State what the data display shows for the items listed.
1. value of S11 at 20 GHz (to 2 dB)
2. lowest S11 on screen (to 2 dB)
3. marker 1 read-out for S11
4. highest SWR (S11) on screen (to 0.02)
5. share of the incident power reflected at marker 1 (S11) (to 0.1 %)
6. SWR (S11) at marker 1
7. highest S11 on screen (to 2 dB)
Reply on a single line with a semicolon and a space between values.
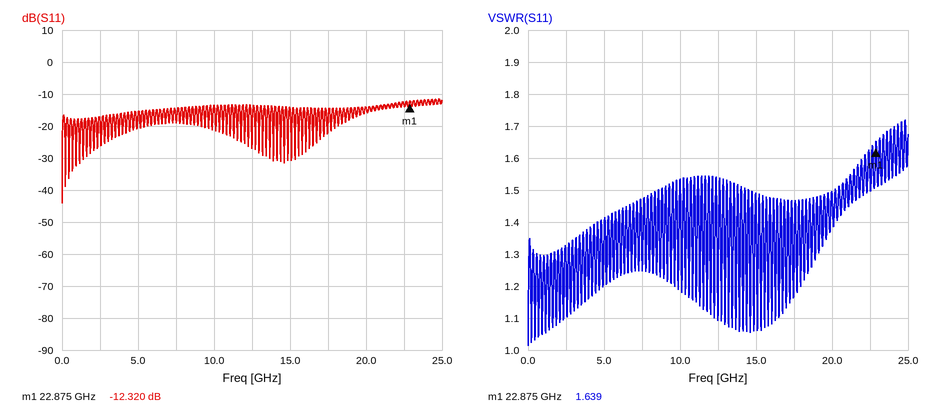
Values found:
-14 dB; -44 dB; -12.320 dB; 1.72; 5.9 %; 1.639; -12 dB
